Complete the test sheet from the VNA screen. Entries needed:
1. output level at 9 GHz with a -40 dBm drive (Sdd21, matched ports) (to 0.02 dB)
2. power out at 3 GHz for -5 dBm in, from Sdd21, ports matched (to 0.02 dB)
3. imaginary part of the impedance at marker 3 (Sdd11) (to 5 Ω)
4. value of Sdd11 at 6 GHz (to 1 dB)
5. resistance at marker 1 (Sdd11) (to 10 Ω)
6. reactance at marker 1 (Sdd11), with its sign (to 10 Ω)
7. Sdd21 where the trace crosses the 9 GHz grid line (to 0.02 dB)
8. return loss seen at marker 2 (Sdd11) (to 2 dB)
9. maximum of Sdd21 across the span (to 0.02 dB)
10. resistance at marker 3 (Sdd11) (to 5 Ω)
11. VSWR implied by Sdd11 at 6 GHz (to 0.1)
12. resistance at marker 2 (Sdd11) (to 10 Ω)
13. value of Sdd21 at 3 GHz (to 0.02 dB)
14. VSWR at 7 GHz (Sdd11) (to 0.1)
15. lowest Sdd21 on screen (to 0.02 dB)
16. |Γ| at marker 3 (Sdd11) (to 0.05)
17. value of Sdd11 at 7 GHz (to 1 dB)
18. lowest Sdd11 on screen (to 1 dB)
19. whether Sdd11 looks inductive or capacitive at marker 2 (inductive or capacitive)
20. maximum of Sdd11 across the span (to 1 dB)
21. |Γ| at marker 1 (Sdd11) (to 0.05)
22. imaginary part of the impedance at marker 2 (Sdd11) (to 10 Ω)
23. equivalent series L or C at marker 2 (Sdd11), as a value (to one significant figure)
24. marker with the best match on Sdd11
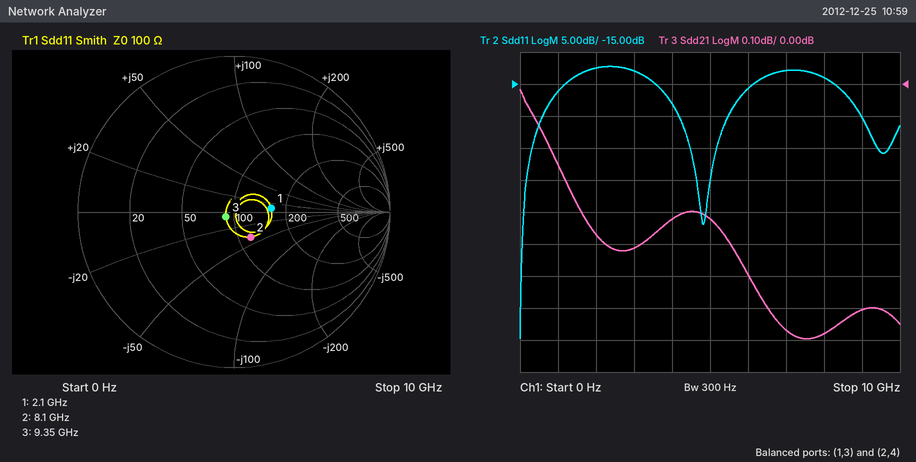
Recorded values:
-40.70 dBm
-5.52 dBm
-5 Ω
-16 dB
160 Ω
+10 Ω
-0.70 dB
14 dB
-0.02 dB
90 Ω
1.4
120 Ω
-0.52 dB
1.6
-0.80 dB
0.05
-13 dB
-55 dB
capacitive
-12 dB
0.25
-40 Ω
500 fF
marker 3
